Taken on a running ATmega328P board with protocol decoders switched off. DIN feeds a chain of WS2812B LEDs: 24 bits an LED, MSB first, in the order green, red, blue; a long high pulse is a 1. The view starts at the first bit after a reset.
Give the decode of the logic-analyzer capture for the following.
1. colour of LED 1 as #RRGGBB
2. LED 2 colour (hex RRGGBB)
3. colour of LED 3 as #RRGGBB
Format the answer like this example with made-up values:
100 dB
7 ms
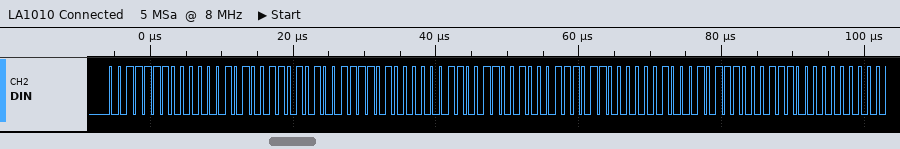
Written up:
#053E35
#033D32
#023B2E
